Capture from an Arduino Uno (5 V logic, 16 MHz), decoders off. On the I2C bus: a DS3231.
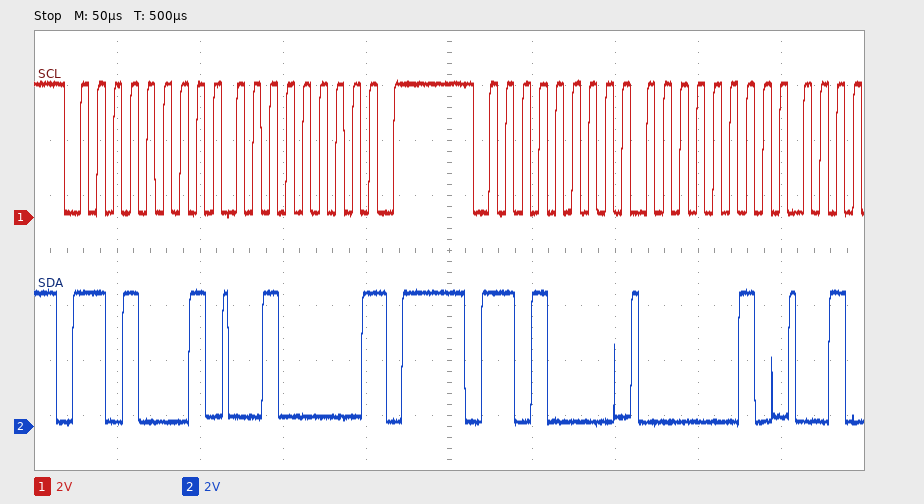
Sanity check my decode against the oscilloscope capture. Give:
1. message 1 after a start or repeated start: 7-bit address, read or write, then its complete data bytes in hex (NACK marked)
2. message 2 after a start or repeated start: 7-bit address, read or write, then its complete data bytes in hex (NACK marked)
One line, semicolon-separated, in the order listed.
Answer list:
0x68 read: 20 NACK; 0x68 write: 02
